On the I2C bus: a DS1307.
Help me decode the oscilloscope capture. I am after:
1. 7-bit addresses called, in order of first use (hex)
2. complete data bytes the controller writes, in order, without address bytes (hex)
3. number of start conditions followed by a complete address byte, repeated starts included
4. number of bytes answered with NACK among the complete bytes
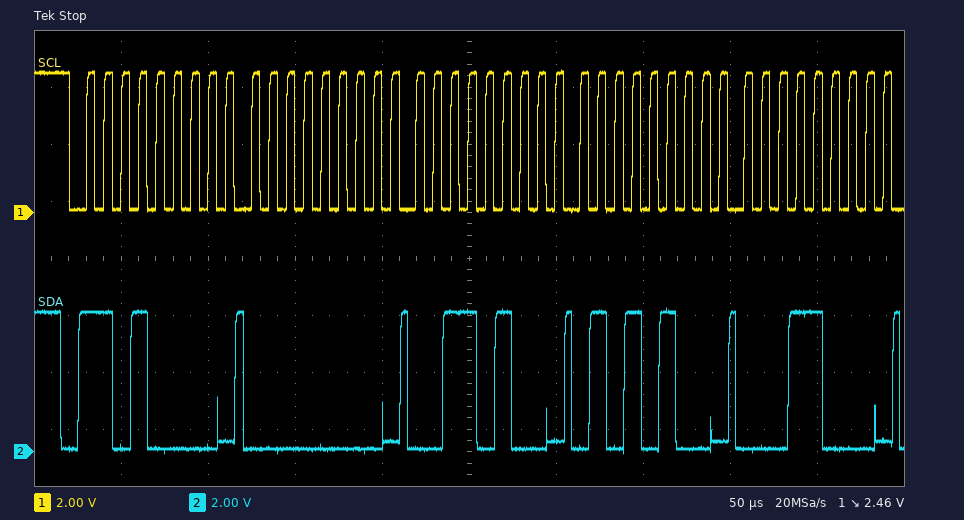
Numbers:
0x68
00 34 54 18
1
0
